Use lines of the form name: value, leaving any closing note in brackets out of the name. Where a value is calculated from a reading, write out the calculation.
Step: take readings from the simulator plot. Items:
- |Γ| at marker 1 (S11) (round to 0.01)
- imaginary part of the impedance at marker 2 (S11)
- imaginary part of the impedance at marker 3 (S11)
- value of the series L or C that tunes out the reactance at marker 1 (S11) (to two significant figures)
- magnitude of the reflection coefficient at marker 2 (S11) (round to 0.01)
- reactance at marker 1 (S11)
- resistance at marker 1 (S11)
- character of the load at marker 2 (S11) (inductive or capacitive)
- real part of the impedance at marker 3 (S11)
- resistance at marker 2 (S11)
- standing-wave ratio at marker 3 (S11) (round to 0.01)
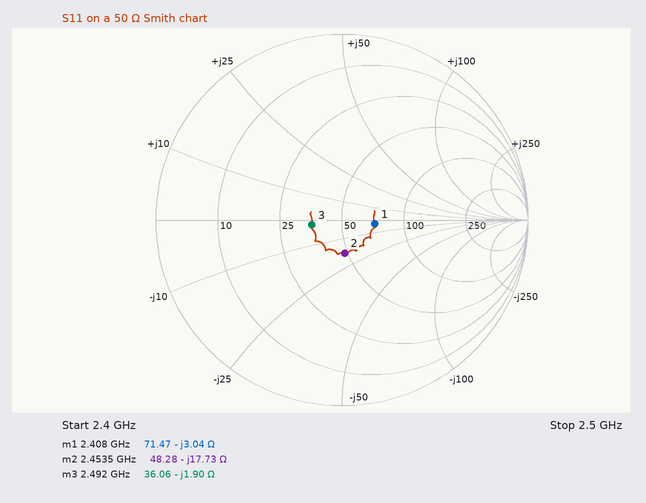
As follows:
|Γ| at marker 1 (S11): 0.18
imaginary part of the impedance at marker 2: -17.73 Ω
imaginary part of the impedance at marker 3: -1.90 Ω
value of the series L or C that tunes out the reactance at marker 1 (S11): L = 3.04 Ω/(2π × 2.408 GHz) ≈ 201 pH, so 200 pH to two significant figures
magnitude of the reflection coefficient at marker 2 (S11): 0.18
reactance at marker 1: -3.04 Ω
resistance at marker 1: 71.47 Ω
character of the load at marker 2 (S11): capacitive
real part of the impedance at marker 3: 36.06 Ω
resistance at marker 2: 48.28 Ω
standing-wave ratio at marker 3 (S11): 1.39
